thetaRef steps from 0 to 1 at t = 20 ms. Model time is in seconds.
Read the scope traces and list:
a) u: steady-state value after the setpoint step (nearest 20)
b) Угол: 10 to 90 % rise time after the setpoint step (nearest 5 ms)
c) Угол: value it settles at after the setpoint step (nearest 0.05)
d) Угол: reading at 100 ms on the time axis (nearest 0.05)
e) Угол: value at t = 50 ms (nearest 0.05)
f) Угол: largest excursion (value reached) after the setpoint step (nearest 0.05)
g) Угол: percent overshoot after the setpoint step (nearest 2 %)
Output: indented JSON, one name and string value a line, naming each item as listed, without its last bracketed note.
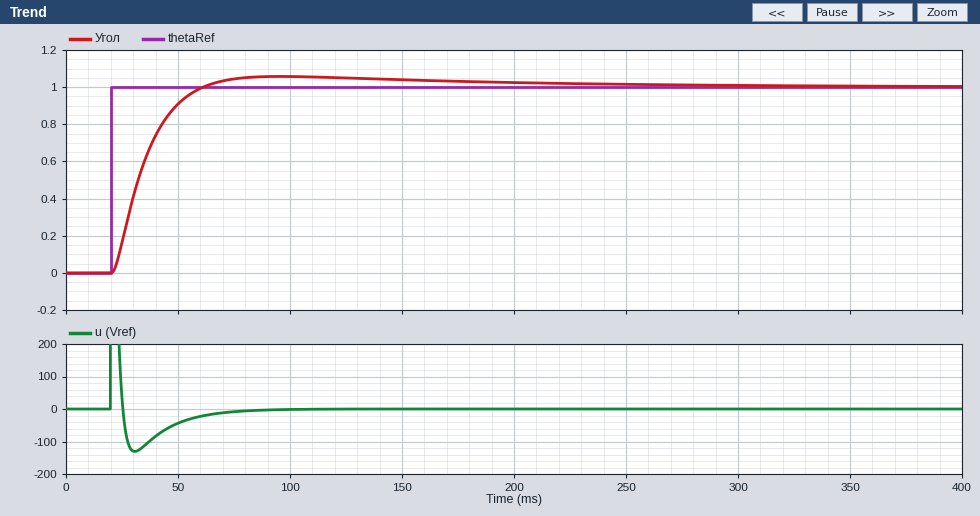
{
  "u: steady-state value after the setpoint step": "0",
  "Угол: 10 to 90 % rise time after the setpoint step": "25 ms",
  "Угол: value it settles at after the setpoint step": "1.00",
  "Угол: reading at 100 ms on the time axis": "1.05",
  "Угол: value at t = 50 ms": "0.90",
  "Угол: largest excursion (value reached) after the setpoint step": "1.05",
  "Угол: percent overshoot after the setpoint step": "6 %"
}
